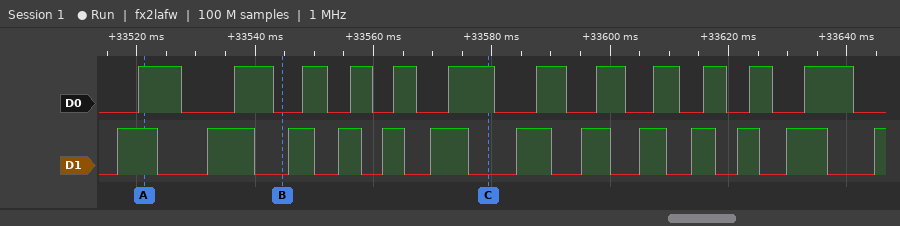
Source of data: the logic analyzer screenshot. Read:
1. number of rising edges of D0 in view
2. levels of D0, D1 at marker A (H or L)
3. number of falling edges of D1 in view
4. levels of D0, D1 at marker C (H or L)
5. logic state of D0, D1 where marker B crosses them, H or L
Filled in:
12
D0=H, D1=H
12
D0=H, D1=L
D0=L, D1=L
